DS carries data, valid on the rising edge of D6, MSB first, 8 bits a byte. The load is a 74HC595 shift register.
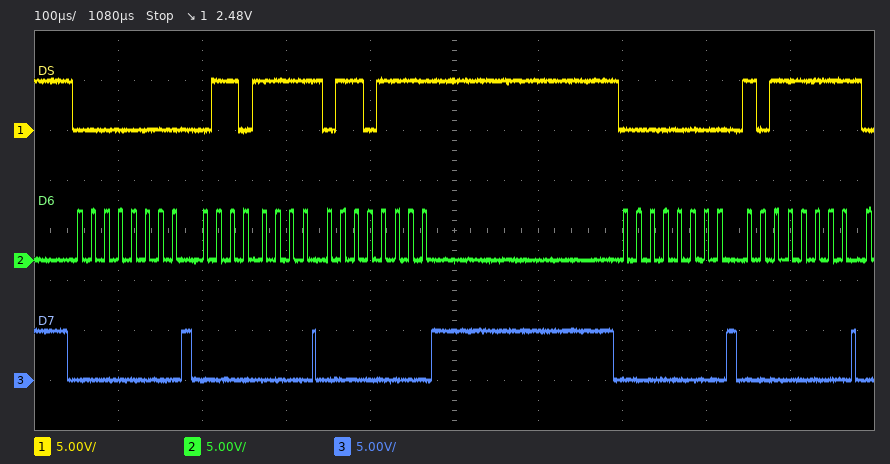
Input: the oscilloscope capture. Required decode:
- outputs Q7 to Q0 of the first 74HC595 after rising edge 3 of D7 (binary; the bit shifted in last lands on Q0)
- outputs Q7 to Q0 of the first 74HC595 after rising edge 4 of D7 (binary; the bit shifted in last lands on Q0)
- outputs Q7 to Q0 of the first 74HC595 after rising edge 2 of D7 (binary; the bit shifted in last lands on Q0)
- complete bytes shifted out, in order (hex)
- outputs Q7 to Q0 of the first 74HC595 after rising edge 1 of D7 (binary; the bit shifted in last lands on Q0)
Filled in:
01101111
00000000
01101111
00 6F 6F 00 BF
00000000
